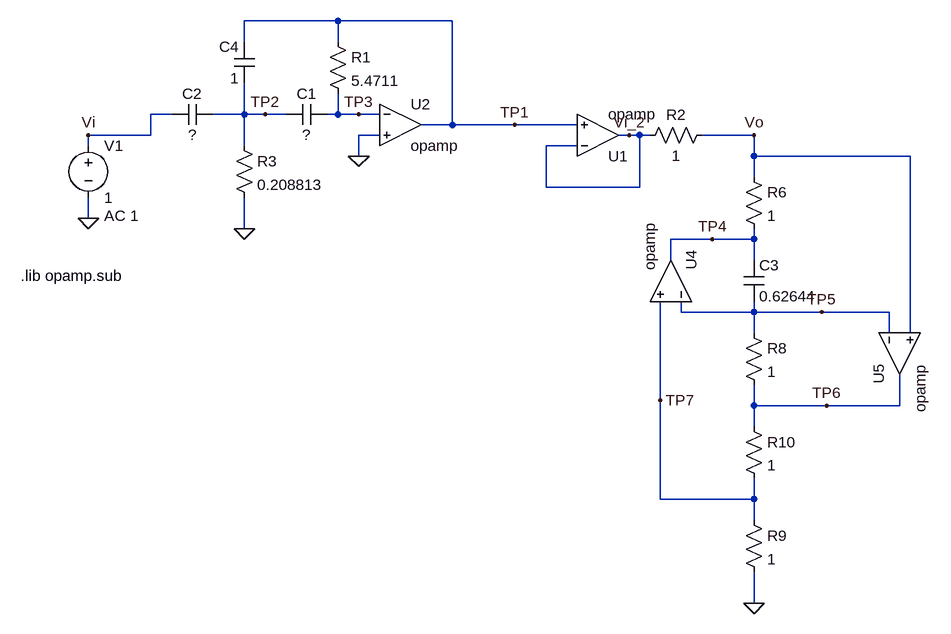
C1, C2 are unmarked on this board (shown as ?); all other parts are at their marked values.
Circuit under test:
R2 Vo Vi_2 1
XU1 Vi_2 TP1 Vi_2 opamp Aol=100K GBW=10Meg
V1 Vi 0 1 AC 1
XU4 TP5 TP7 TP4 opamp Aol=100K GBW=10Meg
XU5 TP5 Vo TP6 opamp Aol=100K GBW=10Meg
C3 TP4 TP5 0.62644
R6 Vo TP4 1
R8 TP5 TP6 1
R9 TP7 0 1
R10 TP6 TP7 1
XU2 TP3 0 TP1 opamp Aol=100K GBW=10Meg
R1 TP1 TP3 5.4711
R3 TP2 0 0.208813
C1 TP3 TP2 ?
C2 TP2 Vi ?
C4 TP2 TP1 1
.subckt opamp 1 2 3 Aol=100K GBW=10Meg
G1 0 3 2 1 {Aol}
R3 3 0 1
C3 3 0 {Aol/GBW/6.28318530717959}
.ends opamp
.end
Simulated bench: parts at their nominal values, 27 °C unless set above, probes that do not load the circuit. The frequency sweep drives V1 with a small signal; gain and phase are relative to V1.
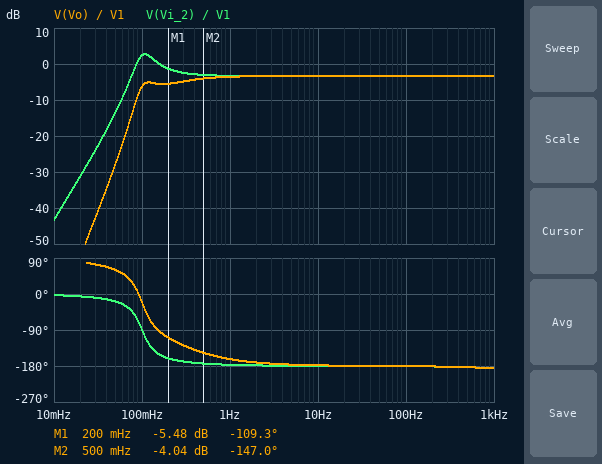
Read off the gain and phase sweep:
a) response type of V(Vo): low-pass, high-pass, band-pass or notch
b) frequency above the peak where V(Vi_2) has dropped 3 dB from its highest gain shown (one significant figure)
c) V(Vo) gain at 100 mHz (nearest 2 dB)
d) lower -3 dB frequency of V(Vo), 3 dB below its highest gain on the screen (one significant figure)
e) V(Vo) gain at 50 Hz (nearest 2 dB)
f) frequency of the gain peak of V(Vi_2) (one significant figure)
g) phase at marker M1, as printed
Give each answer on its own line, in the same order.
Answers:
high-pass
200 mHz
-6 dB
100 mHz
-4 dB
100 mHz
-109.3 deg
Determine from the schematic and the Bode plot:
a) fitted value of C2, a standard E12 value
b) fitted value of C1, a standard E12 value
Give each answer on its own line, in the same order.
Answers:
680 mF
2.2 F
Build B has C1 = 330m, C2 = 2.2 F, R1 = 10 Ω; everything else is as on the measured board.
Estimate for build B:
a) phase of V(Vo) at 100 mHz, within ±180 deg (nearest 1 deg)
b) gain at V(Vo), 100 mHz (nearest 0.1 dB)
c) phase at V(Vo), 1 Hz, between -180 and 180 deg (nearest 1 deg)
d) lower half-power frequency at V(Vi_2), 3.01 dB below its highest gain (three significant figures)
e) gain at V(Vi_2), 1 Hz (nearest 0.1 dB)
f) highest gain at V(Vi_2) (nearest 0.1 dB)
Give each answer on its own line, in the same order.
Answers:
36 deg
-11.9 dB
-156 deg
162 mHz
7.0 dB
8.8 dB
